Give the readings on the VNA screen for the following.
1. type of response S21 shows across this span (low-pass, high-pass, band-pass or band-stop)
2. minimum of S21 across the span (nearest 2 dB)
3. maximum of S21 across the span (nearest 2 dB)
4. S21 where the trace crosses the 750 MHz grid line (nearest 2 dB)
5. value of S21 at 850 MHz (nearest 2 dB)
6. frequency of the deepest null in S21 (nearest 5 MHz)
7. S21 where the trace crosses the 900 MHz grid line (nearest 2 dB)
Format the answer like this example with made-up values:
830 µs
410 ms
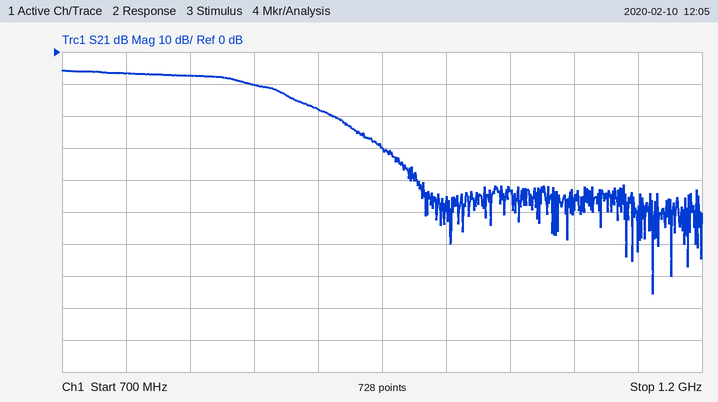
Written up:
low-pass
-76 dB
-6 dB
-6 dB
-10 dB
1.160 GHz
-18 dB
